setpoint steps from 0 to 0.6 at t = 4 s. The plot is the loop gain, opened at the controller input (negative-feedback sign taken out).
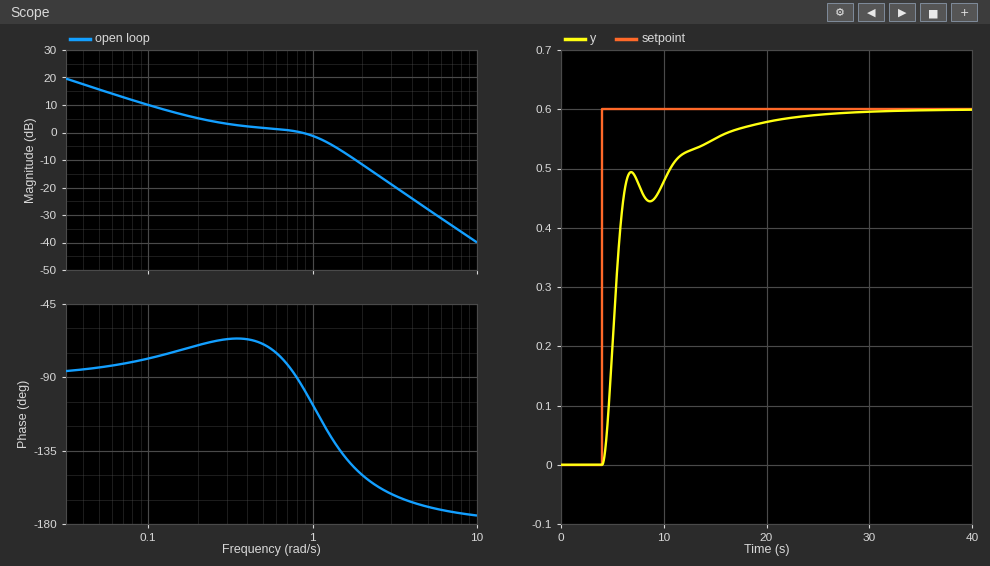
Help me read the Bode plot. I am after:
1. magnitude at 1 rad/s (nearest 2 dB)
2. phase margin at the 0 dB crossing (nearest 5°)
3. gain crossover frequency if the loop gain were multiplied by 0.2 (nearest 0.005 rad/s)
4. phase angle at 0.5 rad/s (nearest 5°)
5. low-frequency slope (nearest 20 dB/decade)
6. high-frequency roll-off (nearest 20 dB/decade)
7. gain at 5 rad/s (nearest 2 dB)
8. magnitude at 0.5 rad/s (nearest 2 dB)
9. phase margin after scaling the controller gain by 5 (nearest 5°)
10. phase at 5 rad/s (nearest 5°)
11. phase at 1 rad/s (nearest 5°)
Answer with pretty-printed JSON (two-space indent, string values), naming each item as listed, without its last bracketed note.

{
  "magnitude at 1 rad/s": "-2 dB",
  "phase margin at the 0 dB crossing": "85°",
  "gain crossover frequency if the loop gain were multiplied by 0.2": "0.060 rad/s",
  "phase angle at 0.5 rad/s": "-70°",
  "low-frequency slope": "-20 dB/decade",
  "high-frequency roll-off": "-40 dB/decade",
  "gain at 5 rad/s": "-28 dB",
  "magnitude at 0.5 rad/s": "2 dB",
  "phase margin after scaling the controller gain by 5": "25°",
  "phase at 5 rad/s": "-170°",
  "phase at 1 rad/s": "-105°"
}
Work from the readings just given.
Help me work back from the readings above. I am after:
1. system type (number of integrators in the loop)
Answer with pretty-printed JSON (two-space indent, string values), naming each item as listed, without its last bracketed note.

{
  "system type": "1"
}
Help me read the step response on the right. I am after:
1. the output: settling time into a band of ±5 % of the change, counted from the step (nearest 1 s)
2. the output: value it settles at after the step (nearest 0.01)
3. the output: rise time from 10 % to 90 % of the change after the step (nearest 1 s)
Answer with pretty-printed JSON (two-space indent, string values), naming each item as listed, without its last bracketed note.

{
  "the output: settling time into a band of ±5 % of the change, counted from the step": "14 s",
  "the output: value it settles at after the step": "0.60",
  "the output: rise time from 10 % to 90 % of the change after the step": "9 s"
}
